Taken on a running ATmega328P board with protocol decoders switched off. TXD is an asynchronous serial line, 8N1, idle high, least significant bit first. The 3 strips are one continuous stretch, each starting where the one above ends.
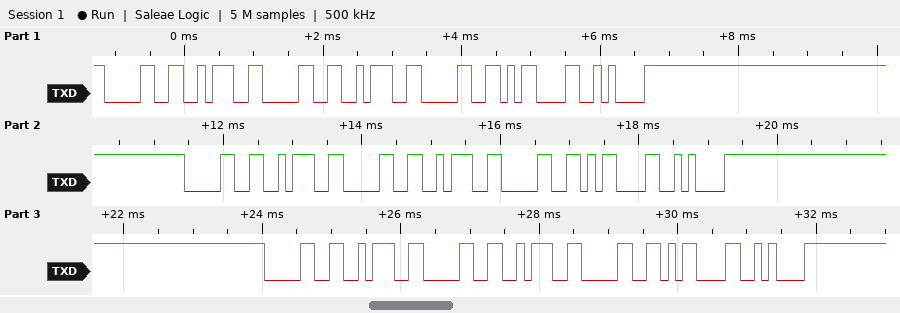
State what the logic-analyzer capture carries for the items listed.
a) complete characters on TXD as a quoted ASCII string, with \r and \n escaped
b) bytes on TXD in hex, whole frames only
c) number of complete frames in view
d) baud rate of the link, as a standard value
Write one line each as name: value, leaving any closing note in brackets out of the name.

complete characters on TXD as a quoted ASCII string, with \r and \n escaped: "0:0:0\r\n0:0:0\r\n0:0:0\r\n"
bytes on TXD in hex, whole frames only: 0x30 0x3A 0x30 0x3A 0x30 0x0D 0x0A 0x30 0x3A 0x30 0x3A 0x30 0x0D 0x0A 0x30 0x3A 0x30 0x3A 0x30 0x0D 0x0A
number of complete frames in view: 21
baud rate of the link, as a standard value: 9600 baud
